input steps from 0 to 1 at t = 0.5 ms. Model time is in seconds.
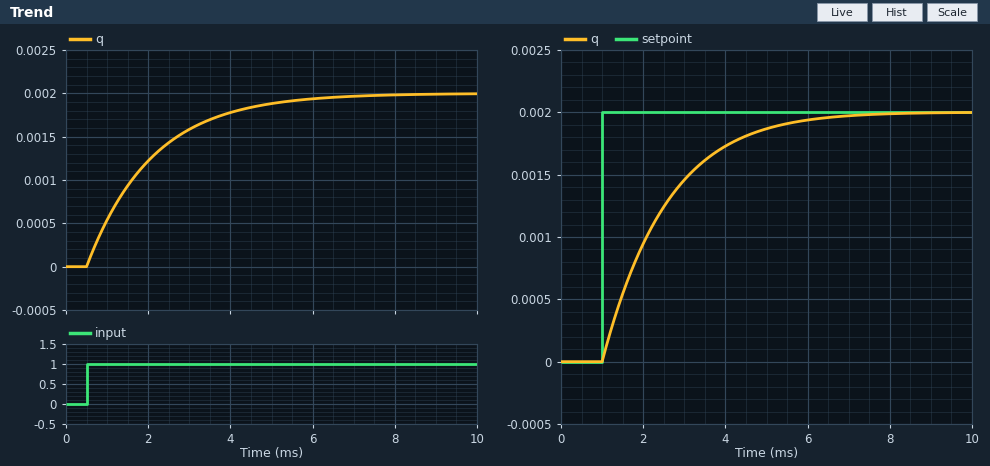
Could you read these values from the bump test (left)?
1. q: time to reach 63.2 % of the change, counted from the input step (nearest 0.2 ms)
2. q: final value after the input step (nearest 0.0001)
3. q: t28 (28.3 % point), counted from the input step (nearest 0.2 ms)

1.6 ms
0.0020
0.6 ms
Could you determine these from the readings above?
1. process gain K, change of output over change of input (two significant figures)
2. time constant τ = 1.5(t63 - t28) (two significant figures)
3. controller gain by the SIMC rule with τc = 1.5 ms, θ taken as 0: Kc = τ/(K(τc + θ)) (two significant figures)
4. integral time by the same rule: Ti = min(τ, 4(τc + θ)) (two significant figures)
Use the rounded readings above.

0.0020
1.5 ms
500
1.5 ms
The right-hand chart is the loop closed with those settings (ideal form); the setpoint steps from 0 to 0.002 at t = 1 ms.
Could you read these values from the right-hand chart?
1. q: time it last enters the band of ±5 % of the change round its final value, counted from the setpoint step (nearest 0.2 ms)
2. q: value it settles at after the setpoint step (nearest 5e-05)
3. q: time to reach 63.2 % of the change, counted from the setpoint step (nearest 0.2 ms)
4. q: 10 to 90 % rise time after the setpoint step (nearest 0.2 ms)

4.4 ms
0.00200
1.6 ms
3.2 ms
